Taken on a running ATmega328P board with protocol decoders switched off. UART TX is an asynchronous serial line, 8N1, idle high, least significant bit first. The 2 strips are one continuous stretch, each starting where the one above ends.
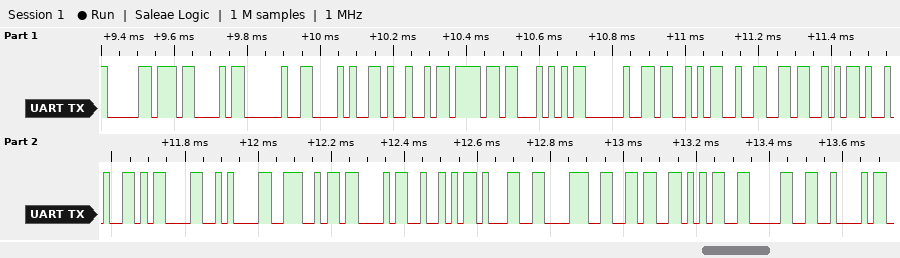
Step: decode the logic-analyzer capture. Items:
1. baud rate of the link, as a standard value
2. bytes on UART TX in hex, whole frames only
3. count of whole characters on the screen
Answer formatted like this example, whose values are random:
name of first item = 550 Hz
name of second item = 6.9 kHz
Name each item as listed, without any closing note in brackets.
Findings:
baud rate of the link, as a standard value = 57600 baud
bytes on UART TX in hex, whole frames only = B0 43 20 28 49 6F 54 20 53 32 53 29 0D 0A 4E 43 52 31 38 36 35 30 42
count of whole characters on the screen = 23
